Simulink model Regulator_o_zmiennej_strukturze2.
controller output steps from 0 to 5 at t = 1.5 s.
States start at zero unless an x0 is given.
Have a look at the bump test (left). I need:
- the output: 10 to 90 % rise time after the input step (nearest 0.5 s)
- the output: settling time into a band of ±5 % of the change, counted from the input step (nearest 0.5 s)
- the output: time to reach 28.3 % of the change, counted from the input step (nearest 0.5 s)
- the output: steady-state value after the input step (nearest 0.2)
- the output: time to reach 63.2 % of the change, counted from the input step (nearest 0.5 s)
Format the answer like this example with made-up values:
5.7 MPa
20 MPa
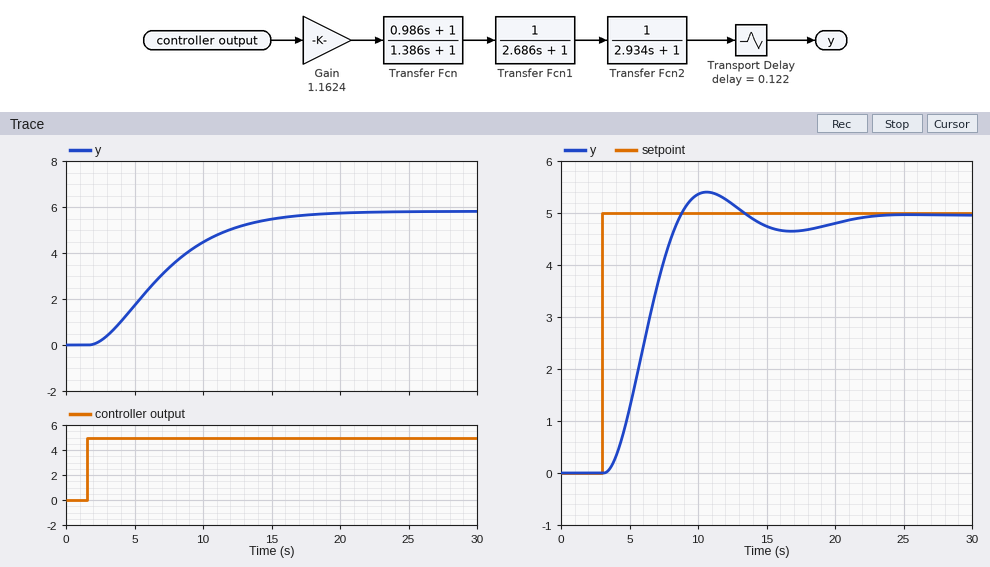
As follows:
10.0 s
14.0 s
3.5 s
5.8
6.5 s
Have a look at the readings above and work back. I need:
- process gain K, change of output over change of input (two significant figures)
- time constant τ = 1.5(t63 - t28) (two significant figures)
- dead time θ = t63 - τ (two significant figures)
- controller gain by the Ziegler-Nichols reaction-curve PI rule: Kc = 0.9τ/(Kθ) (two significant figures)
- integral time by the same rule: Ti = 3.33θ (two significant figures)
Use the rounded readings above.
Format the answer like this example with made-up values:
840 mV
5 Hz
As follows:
1.2
4.5 s
2.0 s
1.7
6.7 s
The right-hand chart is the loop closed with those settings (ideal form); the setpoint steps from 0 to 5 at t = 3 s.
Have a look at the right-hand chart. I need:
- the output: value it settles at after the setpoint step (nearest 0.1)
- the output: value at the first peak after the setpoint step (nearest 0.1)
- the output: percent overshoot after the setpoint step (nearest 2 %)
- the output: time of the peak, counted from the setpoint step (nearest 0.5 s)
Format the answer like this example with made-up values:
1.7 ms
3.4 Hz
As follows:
5.0
5.4
8 %
7.5 s
